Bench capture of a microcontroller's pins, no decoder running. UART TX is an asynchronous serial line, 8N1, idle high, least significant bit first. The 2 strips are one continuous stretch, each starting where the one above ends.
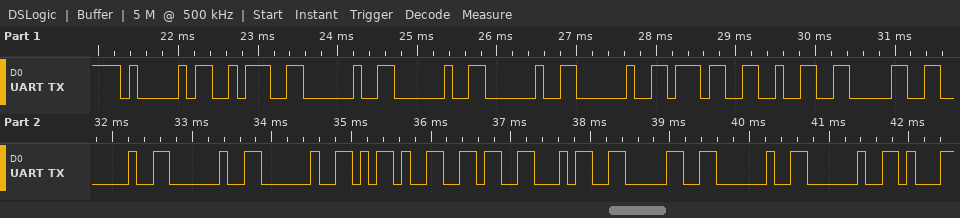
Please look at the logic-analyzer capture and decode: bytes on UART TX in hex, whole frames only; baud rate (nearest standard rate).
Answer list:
0x41 0x3A 0x20 0x20 0x20 0x20 0x37 0x32 0x30 0x20 0x20 0x20 0x2D 0x36 0x34 0x30 0x20 0x20
9600 baud
